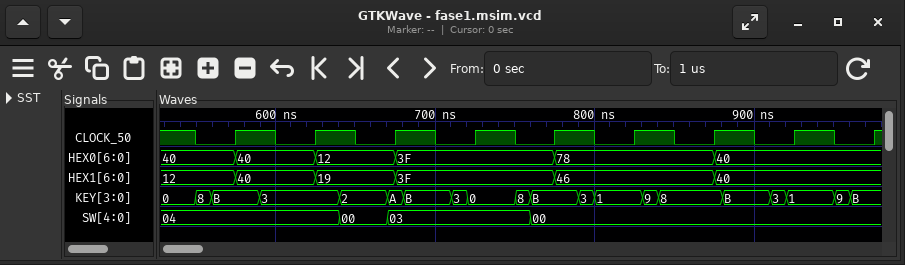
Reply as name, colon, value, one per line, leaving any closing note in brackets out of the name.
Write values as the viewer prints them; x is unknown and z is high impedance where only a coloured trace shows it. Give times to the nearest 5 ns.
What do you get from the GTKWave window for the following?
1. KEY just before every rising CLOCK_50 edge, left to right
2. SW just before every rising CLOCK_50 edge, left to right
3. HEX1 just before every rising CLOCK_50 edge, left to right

KEY just before every rising CLOCK_50 edge, left to right: B, 3, A, 0, B, 1, 8, 1, B
SW just before every rising CLOCK_50 edge, left to right: 04, 04, 03, 03, 00, 00, 00, 00, 00
HEX1 just before every rising CLOCK_50 edge, left to right: 12, 40, 19, 3F, 3F, 46, 46, 40, 40
